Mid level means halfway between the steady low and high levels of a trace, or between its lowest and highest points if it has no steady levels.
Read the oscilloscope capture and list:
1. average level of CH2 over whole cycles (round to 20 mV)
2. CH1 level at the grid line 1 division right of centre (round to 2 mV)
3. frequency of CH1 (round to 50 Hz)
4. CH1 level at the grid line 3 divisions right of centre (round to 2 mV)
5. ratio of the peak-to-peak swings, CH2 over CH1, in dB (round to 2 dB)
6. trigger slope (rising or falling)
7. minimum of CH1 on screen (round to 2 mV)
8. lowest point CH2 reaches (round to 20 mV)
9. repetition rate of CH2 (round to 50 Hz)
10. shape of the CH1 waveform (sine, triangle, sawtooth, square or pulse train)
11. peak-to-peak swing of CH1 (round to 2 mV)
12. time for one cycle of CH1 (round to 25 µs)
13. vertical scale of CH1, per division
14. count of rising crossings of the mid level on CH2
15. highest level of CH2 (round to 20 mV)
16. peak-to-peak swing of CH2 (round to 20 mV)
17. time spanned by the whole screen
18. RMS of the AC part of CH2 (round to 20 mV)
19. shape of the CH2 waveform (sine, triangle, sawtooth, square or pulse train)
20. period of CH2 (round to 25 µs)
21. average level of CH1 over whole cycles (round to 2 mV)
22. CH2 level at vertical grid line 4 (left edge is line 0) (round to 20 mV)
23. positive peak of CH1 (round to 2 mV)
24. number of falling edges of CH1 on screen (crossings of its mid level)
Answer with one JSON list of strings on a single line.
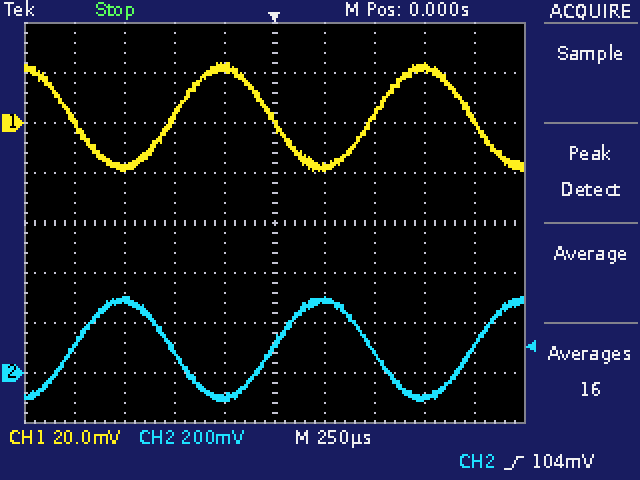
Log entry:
["100 mV", "-18 mV", "1.00 kHz", "22 mV", "20 dB", "rising", "-20 mV", "-120 mV", "1.00 kHz", "sine", "44 mV", "1.000 ms", "20 mV", "3", "300 mV", "420 mV", "2.5 ms", "140 mV", "sine", "1.000 ms", "2 mV", "-100 mV", "24 mV", "3"]
